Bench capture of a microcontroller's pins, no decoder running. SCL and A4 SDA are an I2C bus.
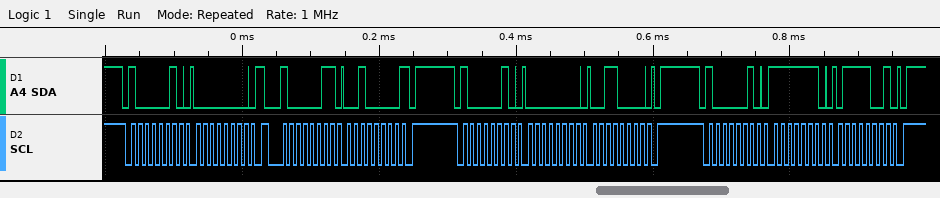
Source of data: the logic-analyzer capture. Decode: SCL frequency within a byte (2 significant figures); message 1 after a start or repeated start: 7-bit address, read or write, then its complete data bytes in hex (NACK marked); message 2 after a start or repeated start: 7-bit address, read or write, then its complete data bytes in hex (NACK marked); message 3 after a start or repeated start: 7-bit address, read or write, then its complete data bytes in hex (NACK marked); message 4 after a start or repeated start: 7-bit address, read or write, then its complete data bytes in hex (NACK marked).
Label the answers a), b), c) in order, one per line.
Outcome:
a) 100 kHz
b) 0x41 write: 00
c) 0x41 read: 20 NACK
d) 0x41 write: 00 30
e) 0x41 write: FE 79
